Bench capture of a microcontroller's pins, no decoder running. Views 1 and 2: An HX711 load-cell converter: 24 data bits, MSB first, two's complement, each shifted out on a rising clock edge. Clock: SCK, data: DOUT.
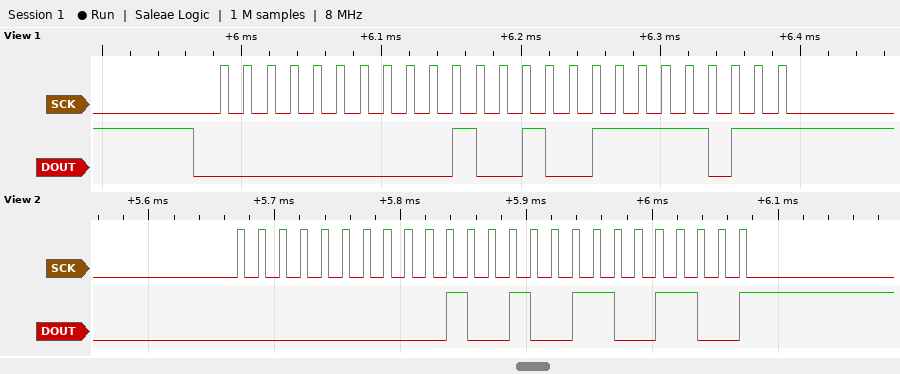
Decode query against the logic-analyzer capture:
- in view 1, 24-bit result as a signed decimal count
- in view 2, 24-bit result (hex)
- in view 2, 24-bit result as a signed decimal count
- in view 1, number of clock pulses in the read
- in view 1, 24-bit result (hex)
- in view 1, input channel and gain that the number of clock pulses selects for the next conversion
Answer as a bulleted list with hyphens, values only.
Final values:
- 9467
- 0x0024CC
- 9420
- 25
- 0x0024FB
- channel A, gain 128
